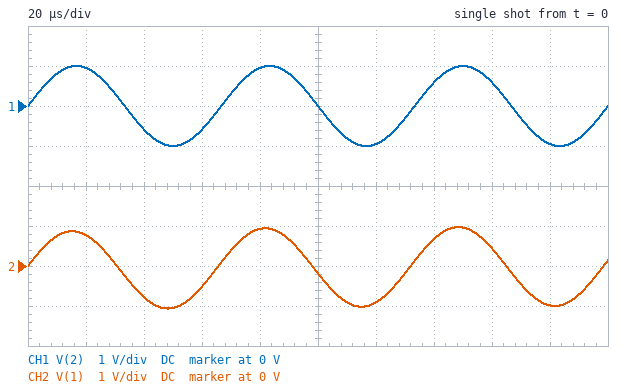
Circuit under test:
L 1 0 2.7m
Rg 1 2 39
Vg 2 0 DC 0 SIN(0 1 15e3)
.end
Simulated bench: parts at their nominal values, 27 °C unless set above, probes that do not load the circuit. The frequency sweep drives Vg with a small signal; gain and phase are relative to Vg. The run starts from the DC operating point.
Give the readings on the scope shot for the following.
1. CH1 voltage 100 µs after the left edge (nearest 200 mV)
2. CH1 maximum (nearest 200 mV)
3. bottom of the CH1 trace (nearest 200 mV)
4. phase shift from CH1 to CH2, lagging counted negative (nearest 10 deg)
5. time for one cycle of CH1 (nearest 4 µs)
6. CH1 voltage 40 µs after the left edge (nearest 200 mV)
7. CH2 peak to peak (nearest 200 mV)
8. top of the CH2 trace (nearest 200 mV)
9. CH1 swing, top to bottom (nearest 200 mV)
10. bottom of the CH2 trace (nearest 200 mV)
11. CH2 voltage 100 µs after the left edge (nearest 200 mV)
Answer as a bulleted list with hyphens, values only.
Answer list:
- 0 V
- 1.0 V
- -1.0 V
- 10 deg
- 68 µs
- -600 mV
- 2.0 V
- 1.0 V
- 2.0 V
- -1.0 V
- -200 mV
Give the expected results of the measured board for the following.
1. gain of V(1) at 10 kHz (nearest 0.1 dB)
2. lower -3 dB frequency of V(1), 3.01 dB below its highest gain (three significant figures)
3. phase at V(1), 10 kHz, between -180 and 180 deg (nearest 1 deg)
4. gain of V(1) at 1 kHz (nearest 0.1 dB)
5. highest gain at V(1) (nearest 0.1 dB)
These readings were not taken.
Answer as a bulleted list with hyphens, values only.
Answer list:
- -0.2 dB
- 2.30 kHz
- 13 deg
- -8.0 dB
- 0 dB
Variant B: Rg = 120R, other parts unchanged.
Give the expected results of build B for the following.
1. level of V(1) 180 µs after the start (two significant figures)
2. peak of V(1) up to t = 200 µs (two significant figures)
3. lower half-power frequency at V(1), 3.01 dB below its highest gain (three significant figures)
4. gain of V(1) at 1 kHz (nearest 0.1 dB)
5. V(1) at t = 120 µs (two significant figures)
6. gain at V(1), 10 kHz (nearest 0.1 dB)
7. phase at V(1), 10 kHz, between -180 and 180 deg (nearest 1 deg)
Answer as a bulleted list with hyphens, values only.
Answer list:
- -900 mV
- 900 mV
- 7.07 kHz
- -17.1 dB
- -660 mV
- -1.8 dB
- 35 deg
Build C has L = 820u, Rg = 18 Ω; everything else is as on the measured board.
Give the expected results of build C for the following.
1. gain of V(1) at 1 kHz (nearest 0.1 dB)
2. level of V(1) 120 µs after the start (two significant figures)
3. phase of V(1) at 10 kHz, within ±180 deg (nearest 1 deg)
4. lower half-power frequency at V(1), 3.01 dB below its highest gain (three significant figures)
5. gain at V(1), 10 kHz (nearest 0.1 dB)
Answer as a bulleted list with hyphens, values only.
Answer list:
- -11.2 dB
- -850 mV
- 19 deg
- 3.49 kHz
- -0.5 dB
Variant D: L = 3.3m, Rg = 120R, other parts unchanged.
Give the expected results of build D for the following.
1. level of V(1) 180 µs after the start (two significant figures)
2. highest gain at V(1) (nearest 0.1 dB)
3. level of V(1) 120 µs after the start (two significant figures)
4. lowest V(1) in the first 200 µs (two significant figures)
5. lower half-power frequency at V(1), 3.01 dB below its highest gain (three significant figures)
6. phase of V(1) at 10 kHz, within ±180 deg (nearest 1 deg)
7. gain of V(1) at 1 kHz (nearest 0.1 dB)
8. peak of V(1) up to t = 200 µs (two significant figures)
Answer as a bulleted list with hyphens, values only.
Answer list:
- -930 mV
- 0 dB
- -730 mV
- -1.0 V
- 5.79 kHz
- 30 deg
- -15.4 dB
- 930 mV
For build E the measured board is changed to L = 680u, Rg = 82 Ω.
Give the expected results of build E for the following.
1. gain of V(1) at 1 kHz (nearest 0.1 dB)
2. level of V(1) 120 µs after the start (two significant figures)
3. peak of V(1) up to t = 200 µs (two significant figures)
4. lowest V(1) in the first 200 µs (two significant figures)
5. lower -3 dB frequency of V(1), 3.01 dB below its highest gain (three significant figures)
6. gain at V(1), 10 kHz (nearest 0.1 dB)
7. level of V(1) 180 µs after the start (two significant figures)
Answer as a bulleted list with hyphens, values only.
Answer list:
- -25.7 dB
- -210 mV
- 620 mV
- -620 mV
- 19.2 kHz
- -6.7 dB
- -510 mV
